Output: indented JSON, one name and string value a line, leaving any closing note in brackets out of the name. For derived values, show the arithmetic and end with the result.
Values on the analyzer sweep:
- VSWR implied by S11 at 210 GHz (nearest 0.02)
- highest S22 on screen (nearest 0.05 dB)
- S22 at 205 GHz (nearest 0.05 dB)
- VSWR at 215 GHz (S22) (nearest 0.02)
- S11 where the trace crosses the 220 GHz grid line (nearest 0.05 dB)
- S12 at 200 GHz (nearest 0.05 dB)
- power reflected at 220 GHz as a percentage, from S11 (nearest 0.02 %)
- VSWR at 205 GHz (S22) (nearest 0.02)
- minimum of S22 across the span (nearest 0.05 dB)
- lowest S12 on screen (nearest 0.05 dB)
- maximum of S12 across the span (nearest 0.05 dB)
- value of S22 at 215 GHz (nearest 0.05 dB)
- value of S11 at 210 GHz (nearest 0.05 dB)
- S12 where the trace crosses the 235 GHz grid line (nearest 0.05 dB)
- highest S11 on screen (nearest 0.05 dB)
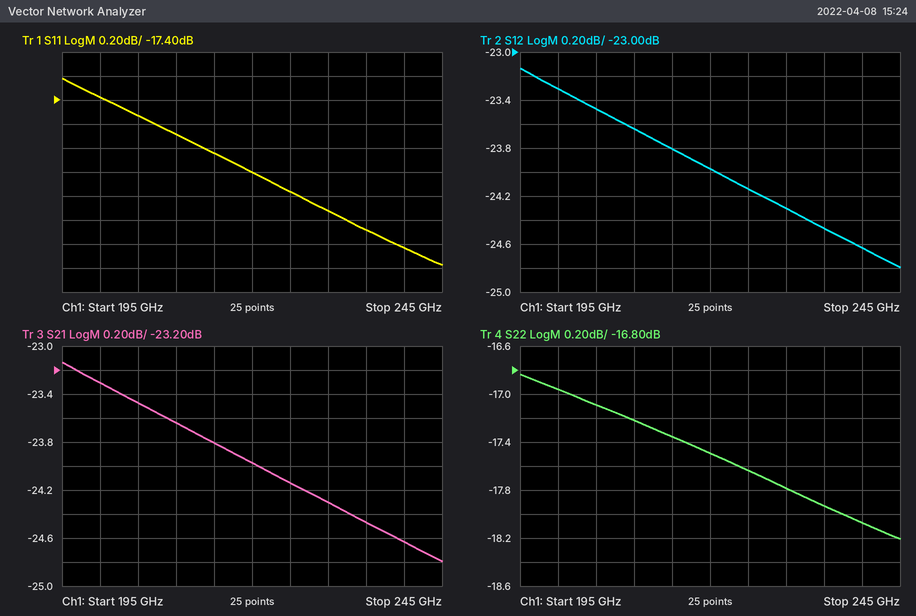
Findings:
{
  "VSWR implied by S11 at 210 GHz": "|Γ| = 10^(-17.7/20) = 0.1303; VSWR = (1 + 0.1303)/(1 − 0.1303) ≈ 1.30",
  "highest S22 on screen": "-16.85 dB",
  "S22 at 205 GHz": "-17.10 dB",
  "VSWR at 215 GHz (S22)": "|Γ| = 10^(-17.35/20) = 0.1357; VSWR = (1 + 0.1357)/(1 − 0.1357) ≈ 1.31, so 1.32 to the nearest 0.02",
  "S11 where the trace crosses the 220 GHz grid line": "-18.00 dB",
  "S12 at 200 GHz": "-23.30 dB",
  "power reflected at 220 GHz as a percentage, from S11": "10^(-18/10) ≈ 1.58 %",
  "VSWR at 205 GHz (S22)": "|Γ| = 10^(-17.1/20) = 0.1396; VSWR = (1 + 0.1396)/(1 − 0.1396) ≈ 1.32",
  "minimum of S22 across the span": "-18.20 dB",
  "lowest S12 on screen": "-24.80 dB",
  "maximum of S12 across the span": "-23.15 dB",
  "value of S22 at 215 GHz": "-17.35 dB",
  "value of S11 at 210 GHz": "-17.70 dB",
  "S12 where the trace crosses the 235 GHz grid line": "-24.45 dB",
  "highest S11 on screen": "-17.20 dB"
}
